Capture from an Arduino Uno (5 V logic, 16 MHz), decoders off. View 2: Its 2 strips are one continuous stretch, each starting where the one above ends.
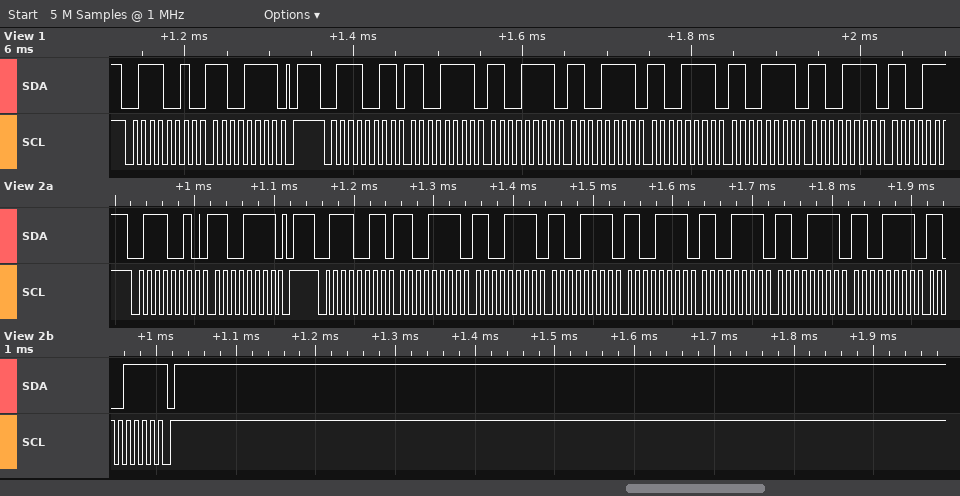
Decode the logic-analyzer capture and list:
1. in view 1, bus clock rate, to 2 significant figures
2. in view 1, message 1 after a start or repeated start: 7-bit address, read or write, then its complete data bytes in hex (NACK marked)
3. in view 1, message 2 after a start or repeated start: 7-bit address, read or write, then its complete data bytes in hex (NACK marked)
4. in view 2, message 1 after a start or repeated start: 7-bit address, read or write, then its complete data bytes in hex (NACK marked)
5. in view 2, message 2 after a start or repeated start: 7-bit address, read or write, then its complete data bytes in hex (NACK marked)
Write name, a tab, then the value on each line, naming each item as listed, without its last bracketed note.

in view 1, bus clock rate, to 2 significant figures	100 kHz
in view 1, message 1 after a start or repeated start: 7-bit address, read or write, then its complete data bytes in hex	0x39 write: CF
in view 1, message 2 after a start or repeated start: 7-bit address, read or write, then its complete data bytes in hex	0x39 read: CF CF CF CF CF CF
in view 2, message 1 after a start or repeated start: 7-bit address, read or write, then its complete data bytes in hex	0x39 write: CF
in view 2, message 2 after a start or repeated start: 7-bit address, read or write, then its complete data bytes in hex	0x39 read: CF CF CF CF CF CF CF CF NACK
